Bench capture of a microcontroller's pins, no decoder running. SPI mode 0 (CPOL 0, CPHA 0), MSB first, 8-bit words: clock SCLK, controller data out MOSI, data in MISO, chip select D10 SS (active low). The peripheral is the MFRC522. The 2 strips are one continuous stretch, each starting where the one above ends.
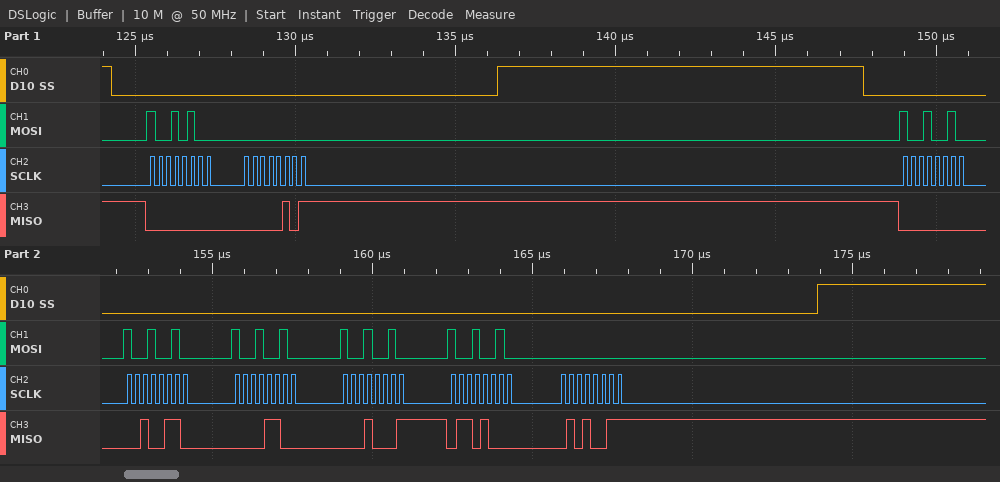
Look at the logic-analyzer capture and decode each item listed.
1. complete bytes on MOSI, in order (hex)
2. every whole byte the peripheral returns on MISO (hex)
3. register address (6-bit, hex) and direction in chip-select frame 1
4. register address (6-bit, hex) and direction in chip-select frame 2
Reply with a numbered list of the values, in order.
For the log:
1. 0x94 0x00 0x92 0x92 0x92 0x92 0x92 0x00
2. 0x00 0x05 0x00 0x26 0x0C 0x11 0x68 0x53
3. 0x0A read
4. 0x09 read
